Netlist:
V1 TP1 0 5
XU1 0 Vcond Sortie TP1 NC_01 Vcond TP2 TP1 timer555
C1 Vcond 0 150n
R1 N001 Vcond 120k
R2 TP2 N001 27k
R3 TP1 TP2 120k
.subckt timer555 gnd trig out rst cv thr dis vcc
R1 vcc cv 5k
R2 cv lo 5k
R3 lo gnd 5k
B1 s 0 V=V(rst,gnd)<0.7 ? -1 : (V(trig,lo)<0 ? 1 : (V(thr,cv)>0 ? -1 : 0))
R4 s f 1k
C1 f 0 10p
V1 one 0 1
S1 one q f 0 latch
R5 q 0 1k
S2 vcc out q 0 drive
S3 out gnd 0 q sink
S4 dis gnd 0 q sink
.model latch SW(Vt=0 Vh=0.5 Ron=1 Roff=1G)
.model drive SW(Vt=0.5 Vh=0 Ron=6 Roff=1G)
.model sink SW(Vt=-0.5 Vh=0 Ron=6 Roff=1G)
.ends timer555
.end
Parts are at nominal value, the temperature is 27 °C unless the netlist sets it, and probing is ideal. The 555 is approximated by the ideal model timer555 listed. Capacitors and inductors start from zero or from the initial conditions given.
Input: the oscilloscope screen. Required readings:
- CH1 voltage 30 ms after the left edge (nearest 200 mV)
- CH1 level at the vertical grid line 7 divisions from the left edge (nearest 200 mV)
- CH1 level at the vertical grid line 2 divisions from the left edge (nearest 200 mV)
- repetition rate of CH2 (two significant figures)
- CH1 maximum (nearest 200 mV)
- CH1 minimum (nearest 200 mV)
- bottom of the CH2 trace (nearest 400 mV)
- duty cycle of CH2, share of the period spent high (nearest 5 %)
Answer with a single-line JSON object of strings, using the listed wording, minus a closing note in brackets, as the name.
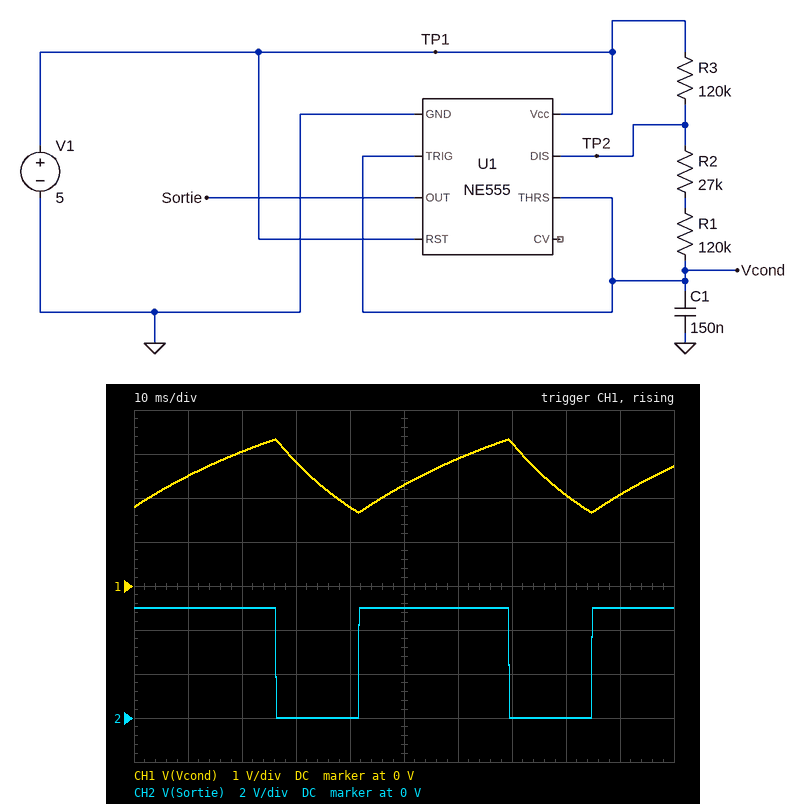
{"CH1 voltage 30 ms after the left edge": "2.8 V", "CH1 level at the vertical grid line 7 divisions from the left edge": "3.2 V", "CH1 level at the vertical grid line 2 divisions from the left edge": "3.0 V", "repetition rate of CH2": "23 Hz", "CH1 maximum": "3.4 V", "CH1 minimum": "1.6 V", "bottom of the CH2 trace": "0 V", "duty cycle of CH2, share of the period spent high": "65 %"}
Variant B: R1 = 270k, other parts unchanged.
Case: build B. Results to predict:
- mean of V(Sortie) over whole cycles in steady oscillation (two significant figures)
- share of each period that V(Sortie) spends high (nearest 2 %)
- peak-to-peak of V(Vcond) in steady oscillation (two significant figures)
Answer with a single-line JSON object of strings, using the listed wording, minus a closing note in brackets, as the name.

{"mean of V(Sortie) over whole cycles in steady oscillation": "2.9 V", "share of each period that V(Sortie) spends high": "58 %", "peak-to-peak of V(Vcond) in steady oscillation": "1.7 V"}
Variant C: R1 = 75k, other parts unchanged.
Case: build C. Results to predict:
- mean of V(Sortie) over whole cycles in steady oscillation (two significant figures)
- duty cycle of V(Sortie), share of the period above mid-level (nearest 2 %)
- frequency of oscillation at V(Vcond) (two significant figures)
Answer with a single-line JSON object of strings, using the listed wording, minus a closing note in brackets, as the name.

{"mean of V(Sortie) over whole cycles in steady oscillation": "3.4 V", "duty cycle of V(Sortie), share of the period above mid-level": "68 %", "frequency of oscillation at V(Vcond)": "30 Hz"}
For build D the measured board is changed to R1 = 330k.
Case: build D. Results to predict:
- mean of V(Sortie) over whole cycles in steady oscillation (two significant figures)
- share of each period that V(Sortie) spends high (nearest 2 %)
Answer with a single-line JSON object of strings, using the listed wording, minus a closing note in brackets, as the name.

{"mean of V(Sortie) over whole cycles in steady oscillation": "2.9 V", "share of each period that V(Sortie) spends high": "58 %"}
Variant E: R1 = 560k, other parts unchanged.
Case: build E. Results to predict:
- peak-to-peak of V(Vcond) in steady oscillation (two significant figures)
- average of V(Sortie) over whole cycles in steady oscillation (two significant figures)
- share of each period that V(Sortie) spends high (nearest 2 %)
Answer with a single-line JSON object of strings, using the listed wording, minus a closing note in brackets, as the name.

{"peak-to-peak of V(Vcond) in steady oscillation": "1.7 V", "average of V(Sortie) over whole cycles in steady oscillation": "2.7 V", "share of each period that V(Sortie) spends high": "54 %"}
